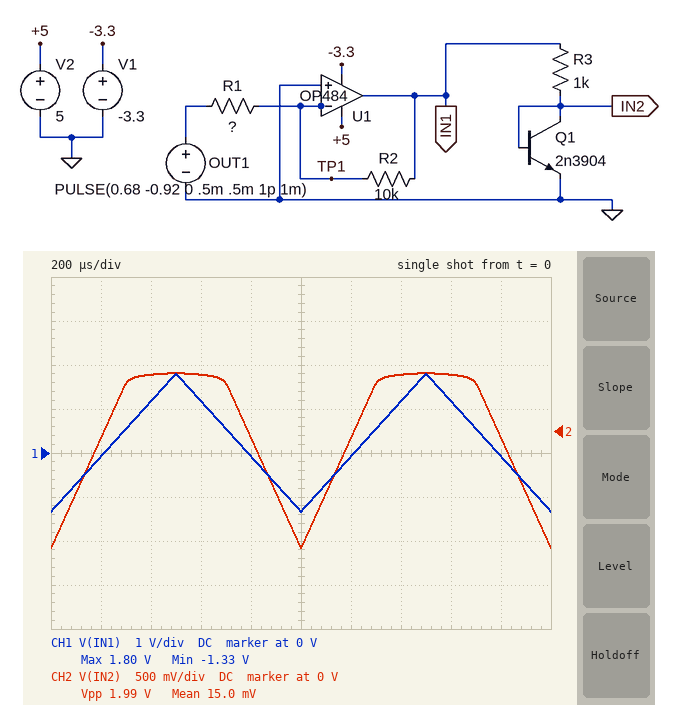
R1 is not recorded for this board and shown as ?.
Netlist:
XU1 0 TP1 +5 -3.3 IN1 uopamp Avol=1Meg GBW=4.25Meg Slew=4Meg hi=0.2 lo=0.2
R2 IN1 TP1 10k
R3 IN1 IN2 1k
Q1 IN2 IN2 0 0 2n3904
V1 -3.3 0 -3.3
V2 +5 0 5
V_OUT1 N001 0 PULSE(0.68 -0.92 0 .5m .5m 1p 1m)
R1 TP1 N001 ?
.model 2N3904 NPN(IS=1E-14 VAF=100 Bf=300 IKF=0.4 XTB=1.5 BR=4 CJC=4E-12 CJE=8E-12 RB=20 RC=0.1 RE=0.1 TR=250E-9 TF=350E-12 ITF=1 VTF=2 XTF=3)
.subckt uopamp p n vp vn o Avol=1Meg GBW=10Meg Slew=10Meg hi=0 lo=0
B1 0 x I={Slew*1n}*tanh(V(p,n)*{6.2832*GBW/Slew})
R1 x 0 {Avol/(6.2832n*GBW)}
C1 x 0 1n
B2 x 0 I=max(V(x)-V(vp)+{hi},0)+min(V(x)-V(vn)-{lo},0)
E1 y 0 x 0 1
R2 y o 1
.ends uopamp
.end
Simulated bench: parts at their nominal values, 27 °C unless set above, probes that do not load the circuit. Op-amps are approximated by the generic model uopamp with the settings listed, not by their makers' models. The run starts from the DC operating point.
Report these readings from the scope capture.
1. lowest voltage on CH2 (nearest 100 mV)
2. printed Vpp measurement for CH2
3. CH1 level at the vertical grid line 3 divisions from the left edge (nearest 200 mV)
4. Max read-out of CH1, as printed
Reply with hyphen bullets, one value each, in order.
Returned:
- -1.3 V
- 1.99 V
- 1.2 V
- 1.80 V
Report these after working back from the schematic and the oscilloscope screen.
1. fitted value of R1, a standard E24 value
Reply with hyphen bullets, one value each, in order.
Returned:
- 5.1 kΩ
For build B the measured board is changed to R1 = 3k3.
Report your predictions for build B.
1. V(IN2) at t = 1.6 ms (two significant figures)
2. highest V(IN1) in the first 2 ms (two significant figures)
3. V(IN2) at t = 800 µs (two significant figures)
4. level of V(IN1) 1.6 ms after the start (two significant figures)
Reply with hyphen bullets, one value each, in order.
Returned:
- 660 mV
- 2.8 V
- -120 mV
- 1.8 V
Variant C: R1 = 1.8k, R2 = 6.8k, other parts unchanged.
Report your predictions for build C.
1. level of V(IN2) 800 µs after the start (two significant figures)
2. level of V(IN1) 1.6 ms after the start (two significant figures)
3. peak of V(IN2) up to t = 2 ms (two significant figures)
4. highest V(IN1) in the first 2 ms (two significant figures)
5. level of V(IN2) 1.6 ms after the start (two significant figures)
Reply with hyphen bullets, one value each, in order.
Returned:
- -150 mV
- 2.3 V
- 680 mV
- 3.5 V
- 670 mV
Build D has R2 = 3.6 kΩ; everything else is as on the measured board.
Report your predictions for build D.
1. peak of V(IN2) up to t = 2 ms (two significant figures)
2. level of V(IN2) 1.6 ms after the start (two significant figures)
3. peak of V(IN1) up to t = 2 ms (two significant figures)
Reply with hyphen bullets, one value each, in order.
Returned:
- 580 mV
- 420 mV
- 650 mV
